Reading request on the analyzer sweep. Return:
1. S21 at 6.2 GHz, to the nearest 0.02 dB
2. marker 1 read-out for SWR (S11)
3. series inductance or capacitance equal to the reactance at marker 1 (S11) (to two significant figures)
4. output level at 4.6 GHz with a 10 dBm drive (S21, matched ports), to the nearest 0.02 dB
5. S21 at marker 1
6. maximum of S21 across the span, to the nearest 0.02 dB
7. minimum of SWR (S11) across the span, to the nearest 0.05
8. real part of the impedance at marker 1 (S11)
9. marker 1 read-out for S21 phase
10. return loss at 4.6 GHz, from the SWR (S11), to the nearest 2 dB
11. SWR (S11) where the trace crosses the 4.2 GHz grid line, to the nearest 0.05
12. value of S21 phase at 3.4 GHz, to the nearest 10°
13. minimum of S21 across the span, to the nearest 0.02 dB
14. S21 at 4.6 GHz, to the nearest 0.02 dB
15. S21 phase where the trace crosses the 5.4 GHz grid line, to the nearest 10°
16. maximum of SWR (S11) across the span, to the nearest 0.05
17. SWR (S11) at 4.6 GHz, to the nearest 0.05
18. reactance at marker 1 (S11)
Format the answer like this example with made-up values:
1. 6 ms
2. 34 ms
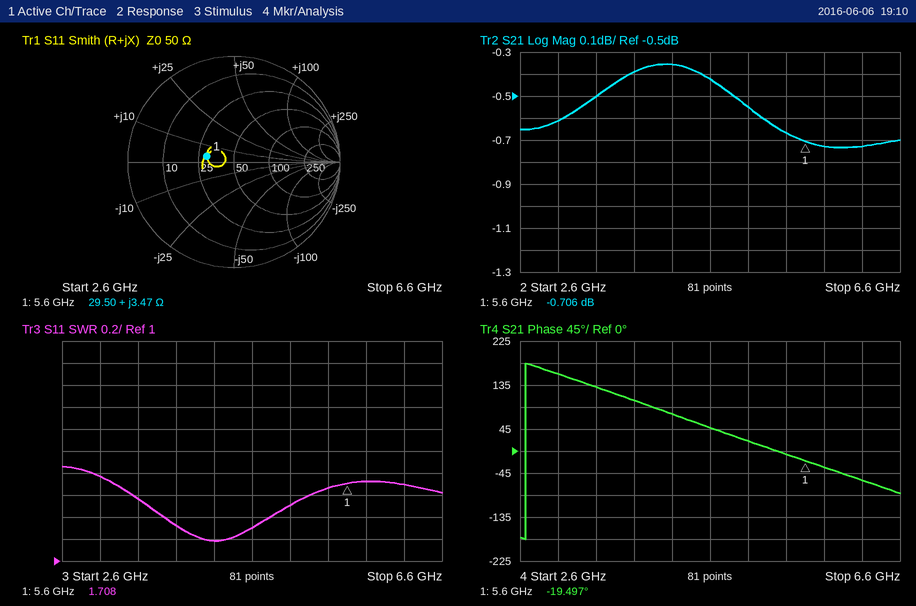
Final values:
1. -0.72 dB
2. 1.708
3. 99 pH
4. 9.58 dBm
5. -0.706 dB
6. -0.36 dB
7. 1.20
8. 29.50 Ω
9. -19.497°
10. 18 dB
11. 1.20
12. 130°
13. -0.74 dB
14. -0.42 dB
15. -10°
16. 1.85
17. 1.30
18. +3.47 Ω
